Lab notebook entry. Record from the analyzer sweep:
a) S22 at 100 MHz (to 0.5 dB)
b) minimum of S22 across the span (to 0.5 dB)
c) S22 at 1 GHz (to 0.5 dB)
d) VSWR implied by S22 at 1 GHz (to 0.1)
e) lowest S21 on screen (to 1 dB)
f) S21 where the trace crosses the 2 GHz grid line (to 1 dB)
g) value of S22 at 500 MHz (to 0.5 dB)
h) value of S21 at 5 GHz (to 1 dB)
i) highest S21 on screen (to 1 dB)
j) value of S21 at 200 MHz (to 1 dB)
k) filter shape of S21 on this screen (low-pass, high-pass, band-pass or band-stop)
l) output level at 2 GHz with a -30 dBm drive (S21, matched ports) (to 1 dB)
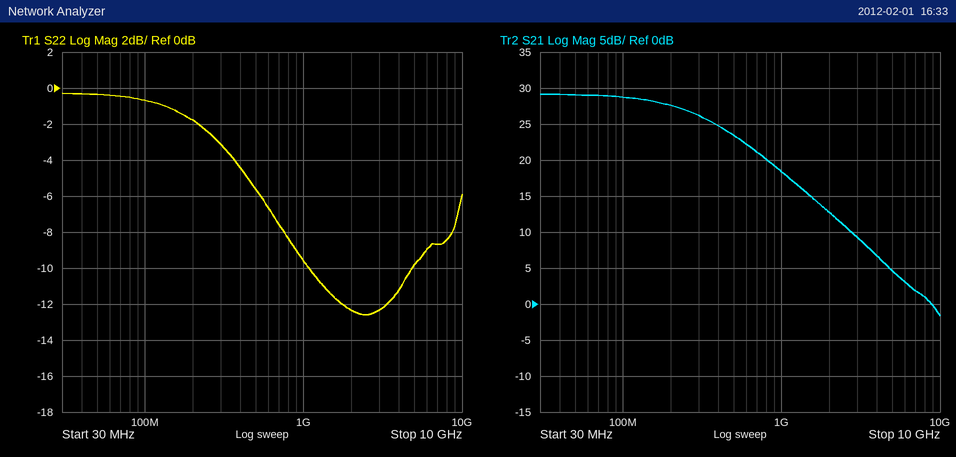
-0.5 dB
-12.5 dB
-9.5 dB
2.0
-2 dB
13 dB
-5.5 dB
5 dB
29 dB
28 dB
low-pass
-17 dBm
